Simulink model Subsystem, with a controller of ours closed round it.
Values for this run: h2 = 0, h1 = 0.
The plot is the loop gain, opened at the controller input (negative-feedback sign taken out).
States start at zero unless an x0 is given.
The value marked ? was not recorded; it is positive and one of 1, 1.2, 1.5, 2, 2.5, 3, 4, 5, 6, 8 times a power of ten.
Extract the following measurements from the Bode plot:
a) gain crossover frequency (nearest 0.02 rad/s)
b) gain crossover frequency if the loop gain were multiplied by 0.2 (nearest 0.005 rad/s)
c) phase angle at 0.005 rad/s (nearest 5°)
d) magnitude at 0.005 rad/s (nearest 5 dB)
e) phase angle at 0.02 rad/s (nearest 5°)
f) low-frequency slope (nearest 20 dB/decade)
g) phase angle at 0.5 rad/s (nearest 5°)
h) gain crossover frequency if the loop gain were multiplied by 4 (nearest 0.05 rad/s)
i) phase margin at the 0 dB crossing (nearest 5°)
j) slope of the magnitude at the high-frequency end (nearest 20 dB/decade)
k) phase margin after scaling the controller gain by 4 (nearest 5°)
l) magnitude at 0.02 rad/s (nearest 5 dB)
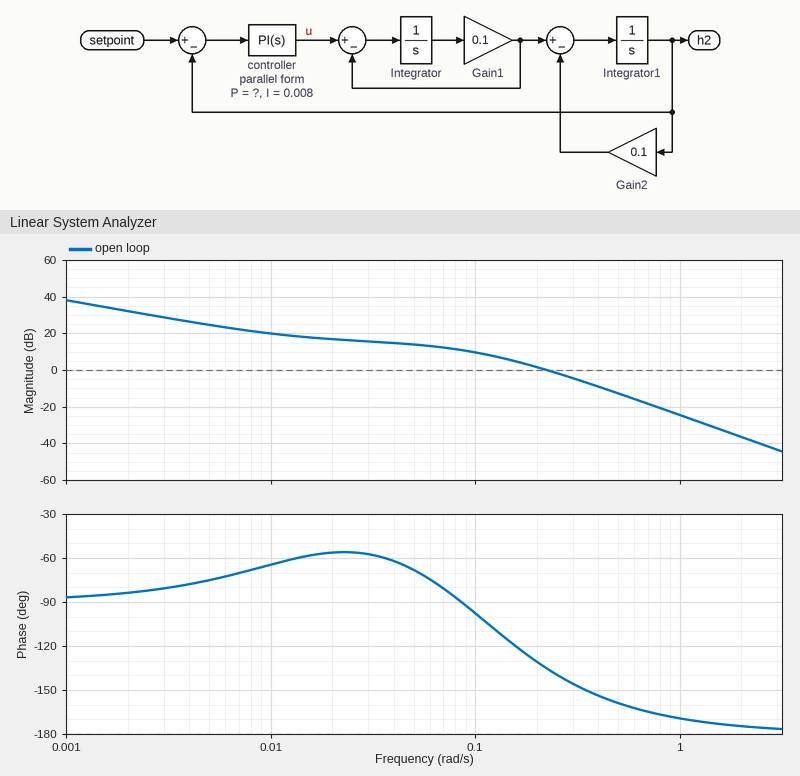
0.22 rad/s
0.050 rad/s
-75°
25 dB
-55°
-20 dB/decade
-160°
0.50 rad/s
45°
-40 dB/decade
20°
15 dB
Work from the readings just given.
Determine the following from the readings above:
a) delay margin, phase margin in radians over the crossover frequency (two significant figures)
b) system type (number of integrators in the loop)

3.6 s
1
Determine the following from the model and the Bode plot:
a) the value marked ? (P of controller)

0.6
